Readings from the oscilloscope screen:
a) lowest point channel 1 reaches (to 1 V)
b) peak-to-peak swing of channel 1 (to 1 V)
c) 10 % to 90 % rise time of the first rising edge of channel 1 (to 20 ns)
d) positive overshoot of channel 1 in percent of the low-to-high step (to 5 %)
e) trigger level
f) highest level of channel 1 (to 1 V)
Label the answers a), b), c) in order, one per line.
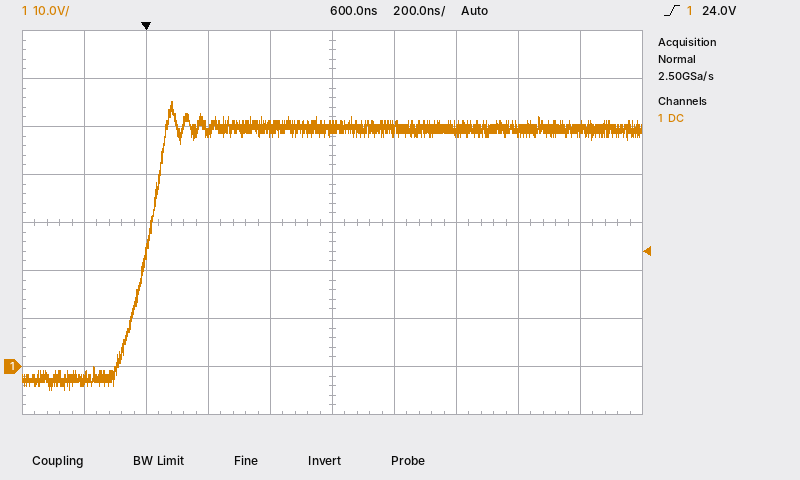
a) -5 V
b) 60 V
c) 140 ns
d) 10 %
e) 24.0 V
f) 55 V
